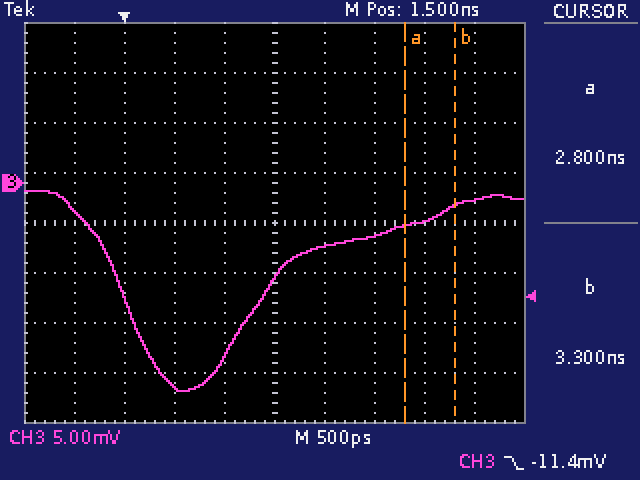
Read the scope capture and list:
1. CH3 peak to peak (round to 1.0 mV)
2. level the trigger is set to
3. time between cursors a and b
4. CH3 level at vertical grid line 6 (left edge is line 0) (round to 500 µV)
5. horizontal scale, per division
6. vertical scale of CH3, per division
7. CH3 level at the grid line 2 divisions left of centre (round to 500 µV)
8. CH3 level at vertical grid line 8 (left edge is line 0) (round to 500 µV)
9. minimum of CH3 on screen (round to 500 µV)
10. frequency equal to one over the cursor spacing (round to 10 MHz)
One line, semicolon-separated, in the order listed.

20.0 mV; -11.4 mV; 500 ps; -6.5 mV; 500 ps; 5 mV; -20.5 mV; -4.0 mV; -21.0 mV; 2.00 GHz
